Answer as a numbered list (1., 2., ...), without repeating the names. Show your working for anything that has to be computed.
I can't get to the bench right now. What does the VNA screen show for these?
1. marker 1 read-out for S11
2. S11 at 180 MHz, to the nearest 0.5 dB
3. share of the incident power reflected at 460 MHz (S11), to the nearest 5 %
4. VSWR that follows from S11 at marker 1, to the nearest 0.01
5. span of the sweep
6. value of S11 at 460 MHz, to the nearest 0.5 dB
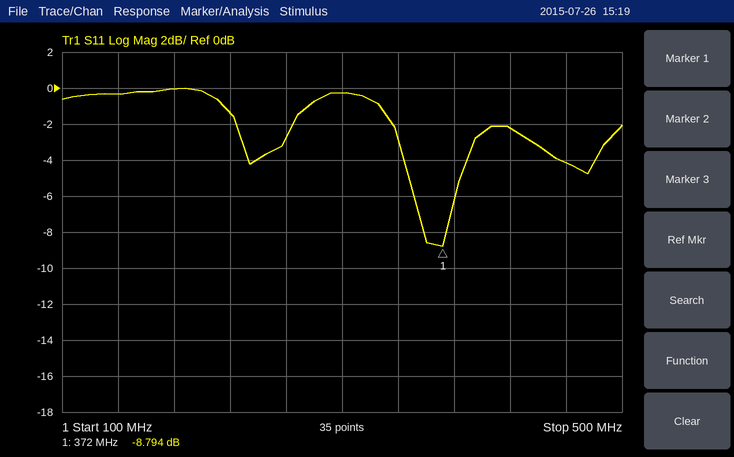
1. -8.794 dB
2. 0.0 dB
3. 10^(-4/10) ≈ 40 %
4. (1 + 0.3633)/(1 − 0.3633) ≈ 2.14
5. 400 MHz
6. -4.0 dB
